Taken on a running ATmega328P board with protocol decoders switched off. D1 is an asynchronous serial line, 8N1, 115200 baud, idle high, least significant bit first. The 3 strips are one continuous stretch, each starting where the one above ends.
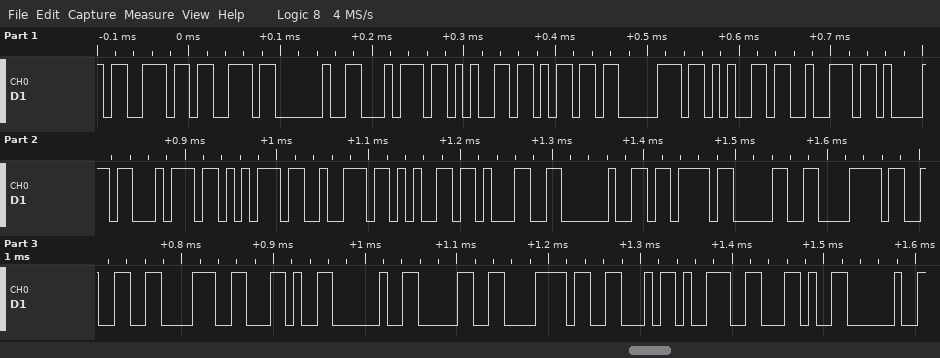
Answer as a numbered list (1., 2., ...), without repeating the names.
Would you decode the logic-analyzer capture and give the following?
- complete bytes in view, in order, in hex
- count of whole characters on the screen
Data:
1. 73 73 20 74 65 6D 70 65 72 61 74 75 72 65 31 20 7B 30 78 32 38 2C 20 30 78 46 39 2C 20
2. 29
